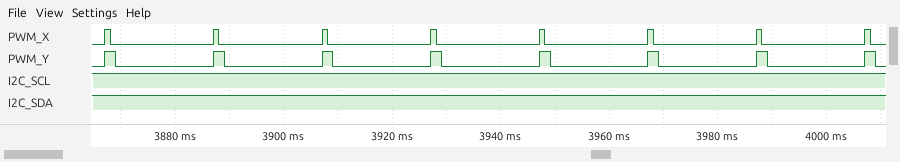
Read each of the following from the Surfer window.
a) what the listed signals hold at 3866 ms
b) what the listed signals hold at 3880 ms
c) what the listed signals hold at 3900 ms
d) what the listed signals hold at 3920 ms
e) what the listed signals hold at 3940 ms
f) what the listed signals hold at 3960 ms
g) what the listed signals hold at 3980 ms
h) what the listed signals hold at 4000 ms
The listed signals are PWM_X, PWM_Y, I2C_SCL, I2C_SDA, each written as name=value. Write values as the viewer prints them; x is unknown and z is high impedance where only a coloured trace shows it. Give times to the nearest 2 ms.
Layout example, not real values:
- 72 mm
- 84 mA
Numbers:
- PWM_X=0, PWM_Y=0, I2C_SCL=1, I2C_SDA=1
- PWM_X=0, PWM_Y=0, I2C_SCL=1, I2C_SDA=1
- PWM_X=0, PWM_Y=0, I2C_SCL=1, I2C_SDA=1
- PWM_X=0, PWM_Y=0, I2C_SCL=1, I2C_SDA=1
- PWM_X=0, PWM_Y=0, I2C_SCL=1, I2C_SDA=1
- PWM_X=0, PWM_Y=0, I2C_SCL=1, I2C_SDA=1
- PWM_X=0, PWM_Y=0, I2C_SCL=1, I2C_SDA=1
- PWM_X=0, PWM_Y=0, I2C_SCL=1, I2C_SDA=1
